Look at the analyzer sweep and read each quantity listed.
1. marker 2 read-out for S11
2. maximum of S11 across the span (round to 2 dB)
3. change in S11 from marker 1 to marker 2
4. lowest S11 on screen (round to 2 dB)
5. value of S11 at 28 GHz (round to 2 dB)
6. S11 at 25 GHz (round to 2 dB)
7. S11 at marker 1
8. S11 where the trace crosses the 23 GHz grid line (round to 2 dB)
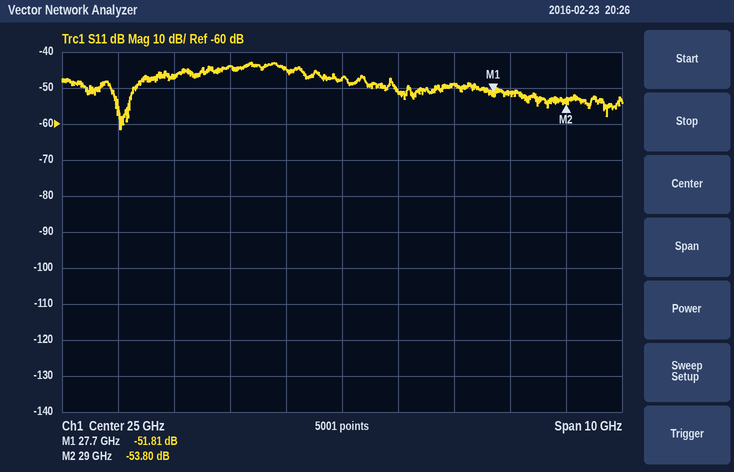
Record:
-53.80 dB
-42 dB
-1.99 dB
-62 dB
-52 dB
-48 dB
-51.81 dB
-44 dB
